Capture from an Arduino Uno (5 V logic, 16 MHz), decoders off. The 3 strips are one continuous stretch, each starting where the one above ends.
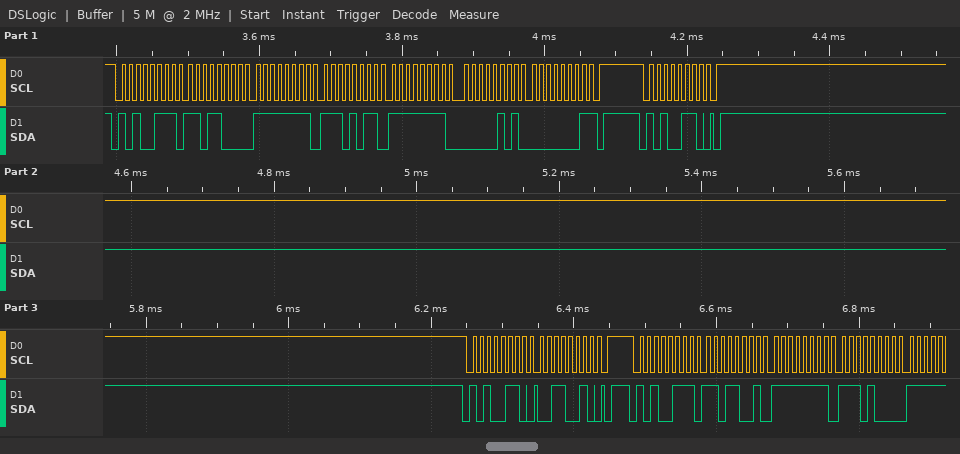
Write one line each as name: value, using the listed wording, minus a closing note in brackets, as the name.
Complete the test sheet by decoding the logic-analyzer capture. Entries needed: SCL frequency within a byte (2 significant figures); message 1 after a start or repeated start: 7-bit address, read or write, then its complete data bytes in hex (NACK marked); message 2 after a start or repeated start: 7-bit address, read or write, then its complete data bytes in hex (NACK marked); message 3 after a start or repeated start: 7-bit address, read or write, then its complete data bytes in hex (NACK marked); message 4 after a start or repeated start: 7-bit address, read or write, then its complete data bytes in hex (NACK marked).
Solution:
SCL frequency within a byte: 100 kHz
message 1 after a start or repeated start: 7-bit address, read or write, then its complete data bytes in hex: 0x53 read: D8 FF EB FF 05 01 NACK
message 2 after a start or repeated start: 7-bit address, read or write, then its complete data bytes in hex: 0x53 write
message 3 after a start or repeated start: 7-bit address, read or write, then its complete data bytes in hex: 0x53 write: 32
message 4 after a start or repeated start: 7-bit address, read or write, then its complete data bytes in hex: 0x53 read: D9 FF E8
